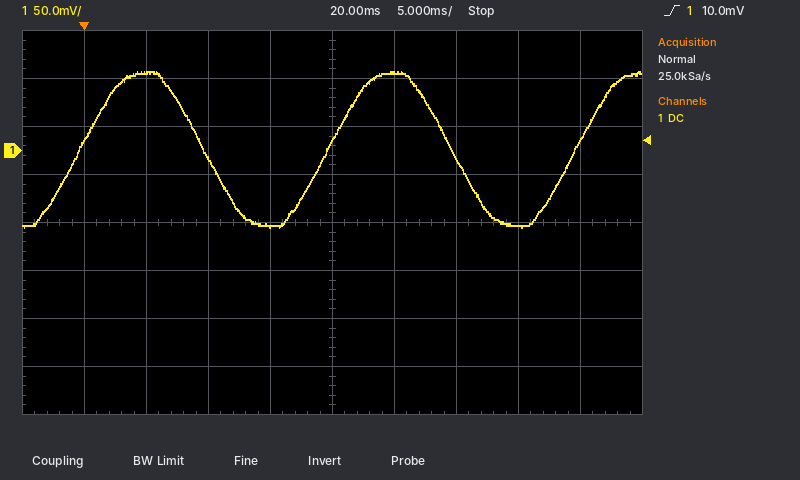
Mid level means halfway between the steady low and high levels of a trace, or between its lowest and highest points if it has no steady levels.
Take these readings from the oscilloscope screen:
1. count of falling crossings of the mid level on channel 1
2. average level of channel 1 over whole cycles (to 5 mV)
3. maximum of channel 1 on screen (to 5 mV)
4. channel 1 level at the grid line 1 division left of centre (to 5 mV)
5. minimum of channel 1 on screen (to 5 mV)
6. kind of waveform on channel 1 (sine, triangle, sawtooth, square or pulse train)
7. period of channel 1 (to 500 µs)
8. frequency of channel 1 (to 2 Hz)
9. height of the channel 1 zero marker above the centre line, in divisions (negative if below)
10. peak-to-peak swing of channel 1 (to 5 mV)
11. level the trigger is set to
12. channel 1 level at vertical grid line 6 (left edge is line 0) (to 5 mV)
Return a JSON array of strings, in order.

["2", "0 mV", "80 mV", "-80 mV", "-80 mV", "sine", "20.0 ms", "50 Hz", "+1.5 div", "160 mV", "10.0 mV", "80 mV"]
